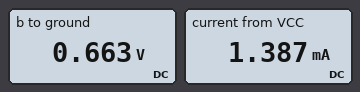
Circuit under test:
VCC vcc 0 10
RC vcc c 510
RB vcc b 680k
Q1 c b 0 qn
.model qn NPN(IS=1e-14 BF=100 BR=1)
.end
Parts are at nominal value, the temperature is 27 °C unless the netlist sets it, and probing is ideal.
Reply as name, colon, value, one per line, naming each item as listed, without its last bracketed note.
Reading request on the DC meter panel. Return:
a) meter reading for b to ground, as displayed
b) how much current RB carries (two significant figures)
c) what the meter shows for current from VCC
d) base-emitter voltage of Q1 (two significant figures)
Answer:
meter reading for b to ground, as displayed: 0.663 V
how much current RB carries: 14 µA
what the meter shows for current from VCC: 1.387 mA
base-emitter voltage of Q1: 660 mV
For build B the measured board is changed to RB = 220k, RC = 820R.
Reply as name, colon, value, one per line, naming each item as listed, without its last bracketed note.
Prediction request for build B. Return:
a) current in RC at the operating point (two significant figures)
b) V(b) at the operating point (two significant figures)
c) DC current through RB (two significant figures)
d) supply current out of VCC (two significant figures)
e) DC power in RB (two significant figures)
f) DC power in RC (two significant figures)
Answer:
current in RC at the operating point: 4.2 mA
V(b) at the operating point: 690 mV
DC current through RB: 42 µA
supply current out of VCC: 4.3 mA
DC power in RB: 390 µW
DC power in RC: 15 mW
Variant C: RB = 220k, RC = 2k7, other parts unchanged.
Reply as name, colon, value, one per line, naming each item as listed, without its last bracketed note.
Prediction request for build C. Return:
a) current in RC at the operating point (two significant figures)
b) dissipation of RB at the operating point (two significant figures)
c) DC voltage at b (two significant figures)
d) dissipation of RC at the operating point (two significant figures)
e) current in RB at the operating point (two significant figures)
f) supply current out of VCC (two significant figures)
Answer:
current in RC at the operating point: 3.6 mA
dissipation of RB at the operating point: 390 µW
DC voltage at b: 690 mV
dissipation of RC at the operating point: 36 mW
current in RB at the operating point: 42 µA
supply current out of VCC: 3.7 mA
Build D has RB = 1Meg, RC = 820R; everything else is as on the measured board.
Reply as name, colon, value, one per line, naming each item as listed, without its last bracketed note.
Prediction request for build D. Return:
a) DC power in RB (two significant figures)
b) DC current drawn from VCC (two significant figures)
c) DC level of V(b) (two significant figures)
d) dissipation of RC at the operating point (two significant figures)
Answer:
DC power in RB: 87 µW
DC current drawn from VCC: 940 µA
DC level of V(b): 650 mV
dissipation of RC at the operating point: 720 µW
